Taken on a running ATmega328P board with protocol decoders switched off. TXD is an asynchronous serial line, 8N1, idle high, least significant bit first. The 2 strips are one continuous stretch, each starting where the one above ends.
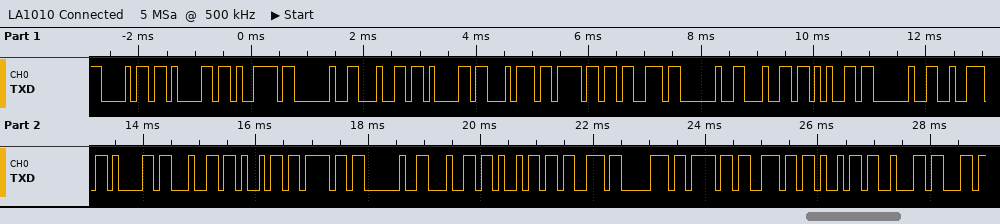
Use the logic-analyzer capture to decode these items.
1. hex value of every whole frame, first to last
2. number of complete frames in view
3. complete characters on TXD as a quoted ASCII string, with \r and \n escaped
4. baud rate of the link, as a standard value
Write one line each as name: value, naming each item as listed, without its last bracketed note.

hex value of every whole frame, first to last: 68 61 79 20 64 61 74 6F 73 20 64 65 20 72 61 64 69 6F 20 64 69 73 70 6F 6E 69 62
number of complete frames in view: 27
complete characters on TXD as a quoted ASCII string, with \r and \n escaped: "hay datos de radio disponib"
baud rate of the link, as a standard value: 9600 baud
